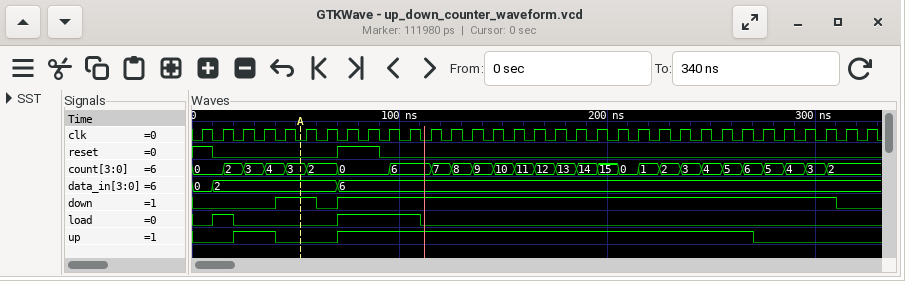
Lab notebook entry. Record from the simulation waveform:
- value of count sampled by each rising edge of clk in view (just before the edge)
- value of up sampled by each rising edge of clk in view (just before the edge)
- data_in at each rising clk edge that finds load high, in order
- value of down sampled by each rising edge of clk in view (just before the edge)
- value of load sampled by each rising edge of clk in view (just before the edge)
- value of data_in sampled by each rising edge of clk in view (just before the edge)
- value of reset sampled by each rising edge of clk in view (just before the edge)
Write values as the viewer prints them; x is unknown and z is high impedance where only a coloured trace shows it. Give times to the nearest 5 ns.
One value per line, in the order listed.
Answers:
0, 0, 2, 3, 4, 3, 2, 0, 0, 0, 6, 6, 7, 8, 9, 10, 11, 12, 13, 14, 15, 0, 1, 2, 3, 4, 5, 6, 5, 4, 3, 2, 2
0 0 1 1 0 0 0 1 1 1 1 1 1 1 1 1 1 1 1 1 1 1 1 1 1 1 1 0 0 0 0 0 0
2, 6, 6, 6, 6
0 0 0 0 1 1 0 1 1 1 1 1 1 1 1 1 1 1 1 1 1 1 1 1 1 1 1 1 1 1 1 0 0
0 1 0 0 0 0 0 1 1 1 1 0 0 0 0 0 0 0 0 0 0 0 0 0 0 0 0 0 0 0 0 0 0
0, 2, 2, 2, 2, 2, 2, 6, 6, 6, 6, 6, 6, 6, 6, 6, 6, 6, 6, 6, 6, 6, 6, 6, 6, 6, 6, 6, 6, 6, 6, 6, 6
1 0 0 0 0 0 0 1 1 0 0 0 0 0 0 0 0 0 0 0 0 0 0 0 0 0 0 0 0 0 0 0 0
